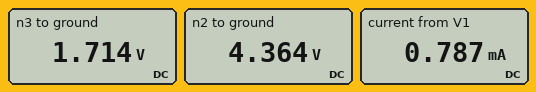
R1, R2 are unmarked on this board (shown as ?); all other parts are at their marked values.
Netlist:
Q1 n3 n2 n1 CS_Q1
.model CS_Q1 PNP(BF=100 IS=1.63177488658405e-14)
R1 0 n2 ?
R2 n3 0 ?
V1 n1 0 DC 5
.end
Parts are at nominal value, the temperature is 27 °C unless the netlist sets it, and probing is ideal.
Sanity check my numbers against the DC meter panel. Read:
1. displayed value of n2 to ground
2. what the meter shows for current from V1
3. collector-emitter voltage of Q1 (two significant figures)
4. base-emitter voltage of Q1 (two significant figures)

4.364 V
0.787 mA
-3.3 V
-640 mV
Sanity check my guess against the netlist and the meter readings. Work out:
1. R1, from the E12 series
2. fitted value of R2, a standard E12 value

560 kΩ
2.2 kΩ
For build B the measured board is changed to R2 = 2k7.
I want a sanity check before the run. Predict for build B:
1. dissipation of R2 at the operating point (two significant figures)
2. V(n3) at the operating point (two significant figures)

1.6 mW
2.1 V
